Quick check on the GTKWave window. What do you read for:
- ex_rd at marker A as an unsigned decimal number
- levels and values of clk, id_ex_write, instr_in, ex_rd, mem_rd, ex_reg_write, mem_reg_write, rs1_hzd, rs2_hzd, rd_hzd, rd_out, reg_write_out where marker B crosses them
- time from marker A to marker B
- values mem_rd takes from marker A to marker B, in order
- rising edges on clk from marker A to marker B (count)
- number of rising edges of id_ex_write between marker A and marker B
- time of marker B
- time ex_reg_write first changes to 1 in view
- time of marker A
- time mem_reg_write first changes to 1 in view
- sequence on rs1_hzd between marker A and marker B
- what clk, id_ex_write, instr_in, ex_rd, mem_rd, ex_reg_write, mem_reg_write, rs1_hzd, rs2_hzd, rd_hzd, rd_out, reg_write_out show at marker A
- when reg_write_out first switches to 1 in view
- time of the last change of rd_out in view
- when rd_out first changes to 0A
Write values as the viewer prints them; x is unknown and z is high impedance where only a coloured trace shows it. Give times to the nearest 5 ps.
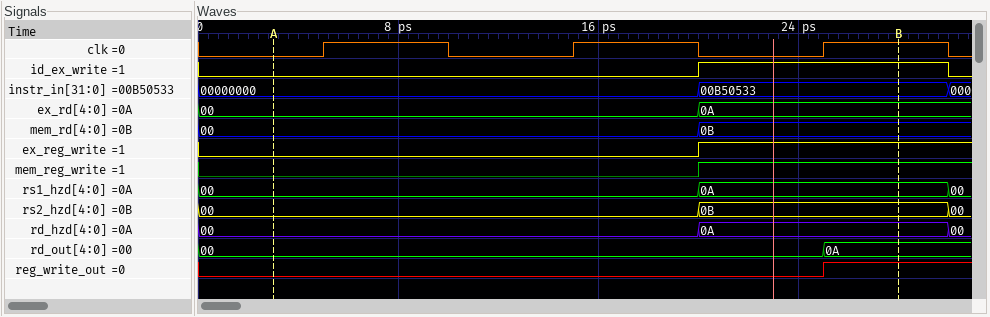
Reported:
0
clk=1, id_ex_write=1, instr_in=00B50533, ex_rd=0A, mem_rd=0B, ex_reg_write=1, mem_reg_write=1, rs1_hzd=0A, rs2_hzd=0B, rd_hzd=0A, rd_out=0A, reg_write_out=1
25 ps
00, 0B
3
1
30 ps
20 ps
5 ps
20 ps
00, 0A
clk=0, id_ex_write=0, instr_in=00000000, ex_rd=00, mem_rd=00, ex_reg_write=0, mem_reg_write=0, rs1_hzd=00, rs2_hzd=00, rd_hzd=00, rd_out=00, reg_write_out=0
25 ps
25 ps
25 ps
